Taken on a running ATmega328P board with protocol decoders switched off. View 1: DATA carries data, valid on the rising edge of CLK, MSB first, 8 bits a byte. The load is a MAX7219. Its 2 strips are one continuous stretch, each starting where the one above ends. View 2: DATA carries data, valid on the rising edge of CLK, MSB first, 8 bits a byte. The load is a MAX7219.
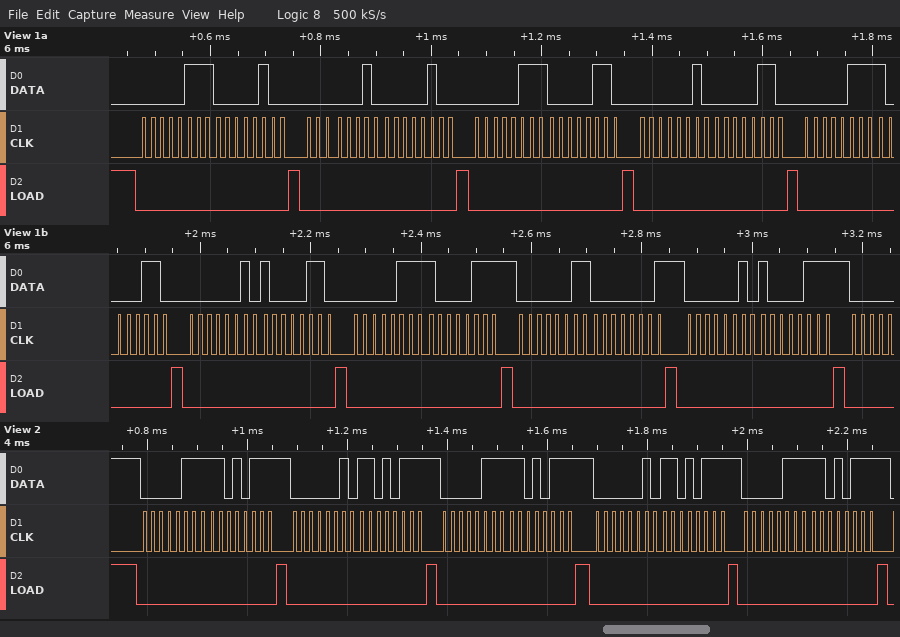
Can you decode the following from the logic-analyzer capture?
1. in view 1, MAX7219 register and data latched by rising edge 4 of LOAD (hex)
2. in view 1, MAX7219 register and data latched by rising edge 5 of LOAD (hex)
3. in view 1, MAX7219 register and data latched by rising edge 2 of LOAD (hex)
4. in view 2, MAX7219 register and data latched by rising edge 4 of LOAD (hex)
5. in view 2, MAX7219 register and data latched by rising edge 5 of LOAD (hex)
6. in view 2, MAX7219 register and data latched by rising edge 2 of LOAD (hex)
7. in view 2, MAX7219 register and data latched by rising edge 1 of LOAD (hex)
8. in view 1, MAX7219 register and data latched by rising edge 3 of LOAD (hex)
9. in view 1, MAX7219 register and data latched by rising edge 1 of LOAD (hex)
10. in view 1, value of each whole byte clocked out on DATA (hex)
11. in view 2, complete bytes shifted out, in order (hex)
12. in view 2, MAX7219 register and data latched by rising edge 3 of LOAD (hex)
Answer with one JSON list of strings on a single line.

["register 0x2, data 0x06", "register 0x7, data 0x86", "register 0x2, data 0x04", "register 0x2, data 0xD7", "register 0x7, data 0xD7", "register 0x2, data 0xD7", "register 0x7, data 0xD7", "register 0x7, data 0x06", "register 0x7, data 0x04", "0x07 0x04 0x02 0x04 0x07 0x06 0x02 0x06 0x07 0x86 0x02 0x86 0x07 0x87 0x03 0x01 0x02 0x87", "07 D7 02 D7 07 D7 02 D7 07 D7", "register 0x7, data 0xD7"]
